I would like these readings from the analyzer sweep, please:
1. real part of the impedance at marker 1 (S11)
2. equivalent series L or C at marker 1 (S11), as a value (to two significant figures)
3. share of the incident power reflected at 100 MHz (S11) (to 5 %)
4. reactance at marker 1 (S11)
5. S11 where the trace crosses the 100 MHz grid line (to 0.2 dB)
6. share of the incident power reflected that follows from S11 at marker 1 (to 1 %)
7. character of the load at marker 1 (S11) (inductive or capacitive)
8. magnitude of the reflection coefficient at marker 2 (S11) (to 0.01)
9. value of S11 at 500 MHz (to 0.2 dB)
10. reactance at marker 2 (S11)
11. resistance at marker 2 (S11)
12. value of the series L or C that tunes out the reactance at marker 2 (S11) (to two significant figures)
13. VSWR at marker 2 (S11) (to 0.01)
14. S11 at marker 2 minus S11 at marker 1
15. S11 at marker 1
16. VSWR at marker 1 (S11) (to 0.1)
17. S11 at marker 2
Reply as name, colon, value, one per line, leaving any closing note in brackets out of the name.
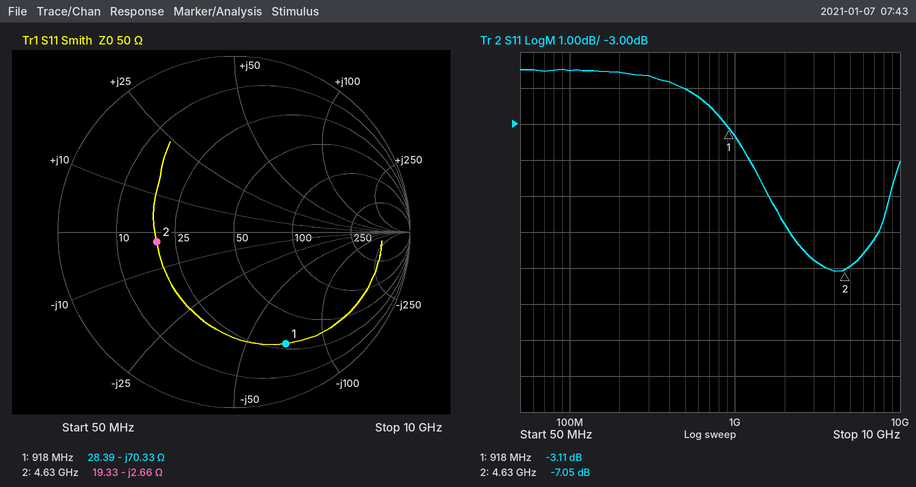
real part of the impedance at marker 1: 28.39 Ω
equivalent series L or C at marker 1 (S11), as a value: 2.5 pF
share of the incident power reflected at 100 MHz (S11): 70 %
reactance at marker 1: -70.33 Ω
S11 where the trace crosses the 100 MHz grid line: -1.6 dB
share of the incident power reflected that follows from S11 at marker 1: 49 %
character of the load at marker 1 (S11): capacitive
magnitude of the reflection coefficient at marker 2 (S11): 0.44
value of S11 at 500 MHz: -2.0 dB
reactance at marker 2: -2.66 Ω
resistance at marker 2: 19.33 Ω
value of the series L or C that tunes out the reactance at marker 2 (S11): 91 pH
VSWR at marker 2 (S11): 2.60
S11 at marker 2 minus S11 at marker 1: -3.94 dB
S11 at marker 1: -3.11 dB
VSWR at marker 1 (S11): 5.6
S11 at marker 2: -7.05 dB
